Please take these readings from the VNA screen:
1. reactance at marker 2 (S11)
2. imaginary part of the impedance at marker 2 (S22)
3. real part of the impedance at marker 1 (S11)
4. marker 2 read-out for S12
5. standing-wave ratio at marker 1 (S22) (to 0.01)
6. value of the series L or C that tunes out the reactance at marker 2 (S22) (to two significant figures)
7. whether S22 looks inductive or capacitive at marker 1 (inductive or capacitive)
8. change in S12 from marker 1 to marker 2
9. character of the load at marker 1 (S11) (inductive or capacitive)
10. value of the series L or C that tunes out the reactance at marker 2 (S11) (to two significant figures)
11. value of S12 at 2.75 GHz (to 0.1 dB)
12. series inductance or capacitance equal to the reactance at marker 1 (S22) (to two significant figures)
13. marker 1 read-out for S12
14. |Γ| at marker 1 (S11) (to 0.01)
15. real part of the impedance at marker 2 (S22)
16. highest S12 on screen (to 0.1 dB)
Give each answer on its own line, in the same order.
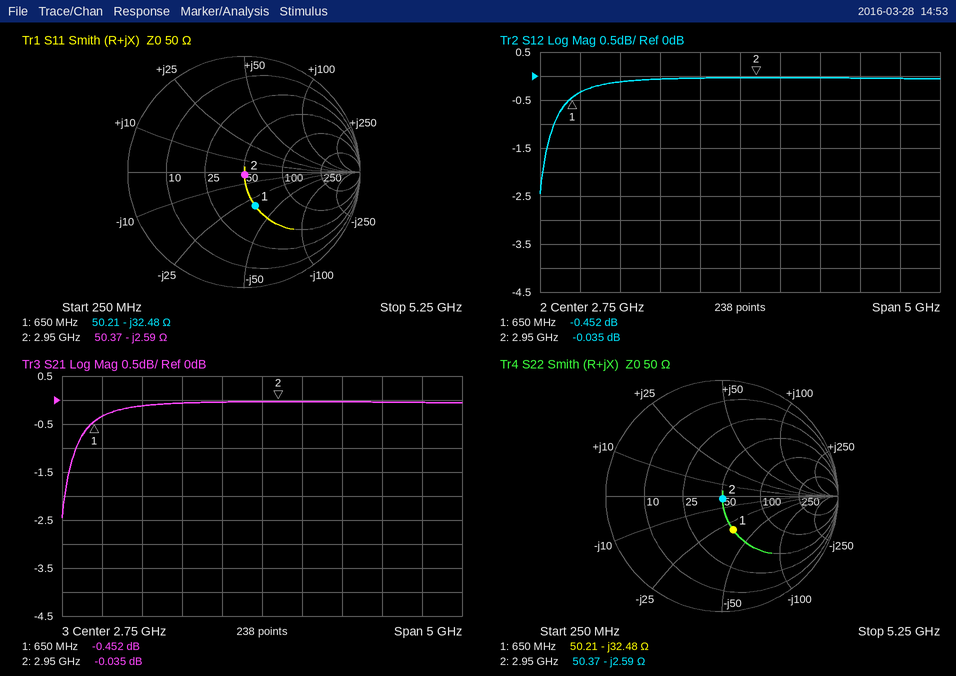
-2.59 Ω
-2.59 Ω
50.21 Ω
-0.035 dB
1.89
140 pH
capacitive
0.417 dB
capacitive
140 pH
0.0 dB
7.5 pF
-0.452 dB
0.31
50.37 Ω
0.0 dB
